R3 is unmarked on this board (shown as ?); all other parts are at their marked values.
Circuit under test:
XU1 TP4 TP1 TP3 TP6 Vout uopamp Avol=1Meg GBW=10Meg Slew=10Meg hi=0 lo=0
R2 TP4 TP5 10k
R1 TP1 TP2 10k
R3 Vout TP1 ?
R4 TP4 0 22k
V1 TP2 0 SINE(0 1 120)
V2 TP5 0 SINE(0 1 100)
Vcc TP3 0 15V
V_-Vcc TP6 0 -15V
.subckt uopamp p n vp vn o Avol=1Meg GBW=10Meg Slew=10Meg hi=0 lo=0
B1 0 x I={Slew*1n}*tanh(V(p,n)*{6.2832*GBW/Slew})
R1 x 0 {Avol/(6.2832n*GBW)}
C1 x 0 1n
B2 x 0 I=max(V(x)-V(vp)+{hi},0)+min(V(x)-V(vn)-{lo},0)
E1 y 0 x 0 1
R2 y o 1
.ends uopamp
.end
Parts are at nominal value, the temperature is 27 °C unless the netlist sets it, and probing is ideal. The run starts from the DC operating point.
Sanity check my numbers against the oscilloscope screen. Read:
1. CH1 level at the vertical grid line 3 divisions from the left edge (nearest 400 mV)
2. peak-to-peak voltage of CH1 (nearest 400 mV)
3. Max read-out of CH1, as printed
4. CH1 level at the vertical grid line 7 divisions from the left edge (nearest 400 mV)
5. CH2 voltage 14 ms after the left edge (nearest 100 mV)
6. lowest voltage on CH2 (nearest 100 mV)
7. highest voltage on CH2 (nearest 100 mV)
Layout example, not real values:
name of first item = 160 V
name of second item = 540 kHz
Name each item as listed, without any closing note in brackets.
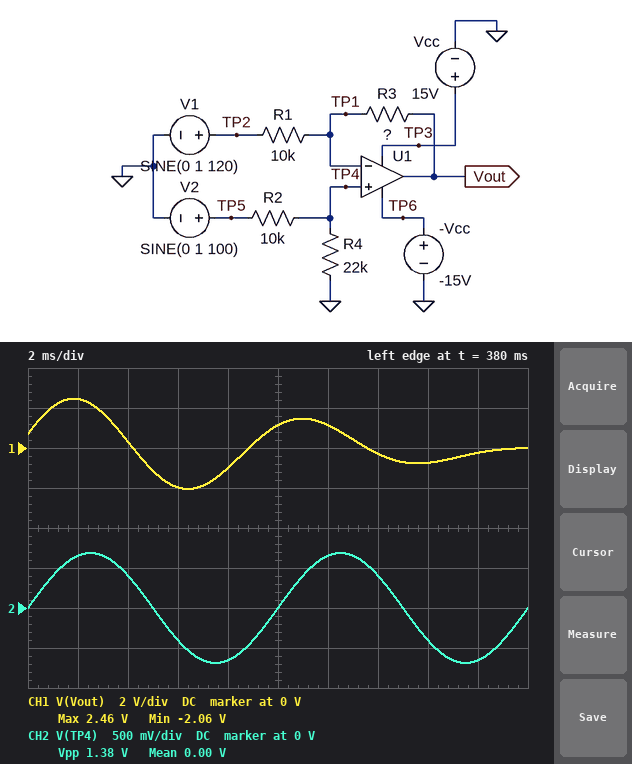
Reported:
CH1 level at the vertical grid line 3 divisions from the left edge = -2.0 V
peak-to-peak voltage of CH1 = 4.4 V
Max read-out of CH1, as printed = 2.46 V
CH1 level at the vertical grid line 7 divisions from the left edge = -400 mV
CH2 voltage 14 ms after the left edge = 400 mV
lowest voltage on CH2 = -700 mV
highest voltage on CH2 = 700 mV
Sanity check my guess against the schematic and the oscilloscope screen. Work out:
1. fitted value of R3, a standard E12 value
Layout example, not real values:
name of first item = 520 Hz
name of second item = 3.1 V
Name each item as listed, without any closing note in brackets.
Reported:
fitted value of R3, a standard E12 value = 12 kΩ
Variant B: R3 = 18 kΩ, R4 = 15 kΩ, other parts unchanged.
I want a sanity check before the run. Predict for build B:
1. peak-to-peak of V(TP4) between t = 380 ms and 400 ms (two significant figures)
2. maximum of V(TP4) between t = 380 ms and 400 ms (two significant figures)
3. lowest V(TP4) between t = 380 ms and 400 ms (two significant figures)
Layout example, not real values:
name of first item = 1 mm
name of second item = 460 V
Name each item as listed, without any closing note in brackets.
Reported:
peak-to-peak of V(TP4) between t = 380 ms and 400 ms = 1.2 V
maximum of V(TP4) between t = 380 ms and 400 ms = 600 mV
lowest V(TP4) between t = 380 ms and 400 ms = -600 mV
